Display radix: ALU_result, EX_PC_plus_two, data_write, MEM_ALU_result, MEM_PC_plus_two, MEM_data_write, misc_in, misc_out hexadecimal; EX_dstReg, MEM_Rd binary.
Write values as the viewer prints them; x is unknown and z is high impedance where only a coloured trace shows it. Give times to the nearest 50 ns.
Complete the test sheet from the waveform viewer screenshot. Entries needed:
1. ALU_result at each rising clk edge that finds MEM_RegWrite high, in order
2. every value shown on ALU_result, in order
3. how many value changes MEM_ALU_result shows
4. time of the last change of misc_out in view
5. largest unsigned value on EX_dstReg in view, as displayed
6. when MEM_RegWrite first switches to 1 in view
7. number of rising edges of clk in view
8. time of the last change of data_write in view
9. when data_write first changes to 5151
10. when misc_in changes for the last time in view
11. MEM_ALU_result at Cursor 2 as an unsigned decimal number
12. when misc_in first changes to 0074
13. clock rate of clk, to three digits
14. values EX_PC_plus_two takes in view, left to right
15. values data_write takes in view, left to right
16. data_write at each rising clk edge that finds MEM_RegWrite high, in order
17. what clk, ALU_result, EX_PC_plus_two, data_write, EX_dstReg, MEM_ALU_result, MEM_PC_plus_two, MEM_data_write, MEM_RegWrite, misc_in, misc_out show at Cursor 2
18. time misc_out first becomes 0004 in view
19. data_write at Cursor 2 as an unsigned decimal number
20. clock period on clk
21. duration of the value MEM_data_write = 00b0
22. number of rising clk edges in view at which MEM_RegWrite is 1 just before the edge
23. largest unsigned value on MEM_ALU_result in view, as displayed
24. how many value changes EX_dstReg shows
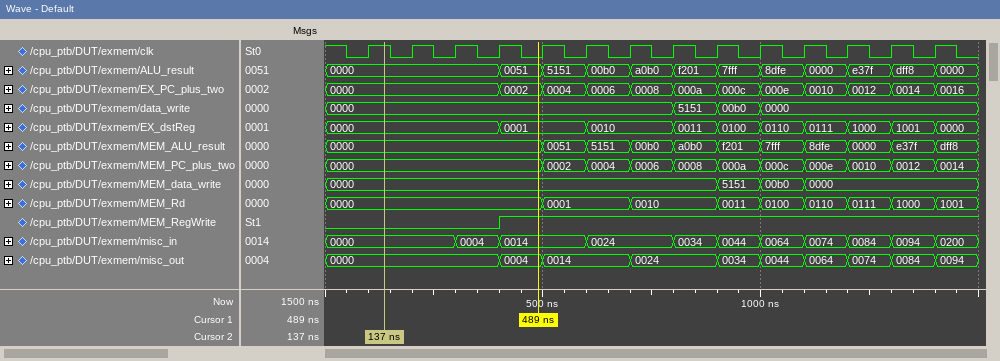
0051, 5151, 00b0, a0b0, f201, 7fff, 8dfe, 0000, e37f, dff8
0000, 0051, 5151, 00b0, a0b0, f201, 7fff, 8dfe, 0000, e37f, dff8, 0000
10
1400 ns
1001
400 ns
14
1000 ns
800 ns
1400 ns
0
1100 ns
10.0 MHz
0000, 0002, 0004, 0006, 0008, 000a, 000c, 000e, 0010, 0012, 0014, 0016
0000, 5151, 00b0, 0000
0000, 0000, 0000, 0000, 5151, 00b0, 0000, 0000, 0000, 0000
clk=1, ALU_result=0000, EX_PC_plus_two=0000, data_write=0000, EX_dstReg=0000, MEM_ALU_result=0000, MEM_PC_plus_two=0000, MEM_data_write=0000, MEM_RegWrite=0, misc_in=0000, misc_out=0000
400 ns
0
100 ns
100 ns
10
f201
9
